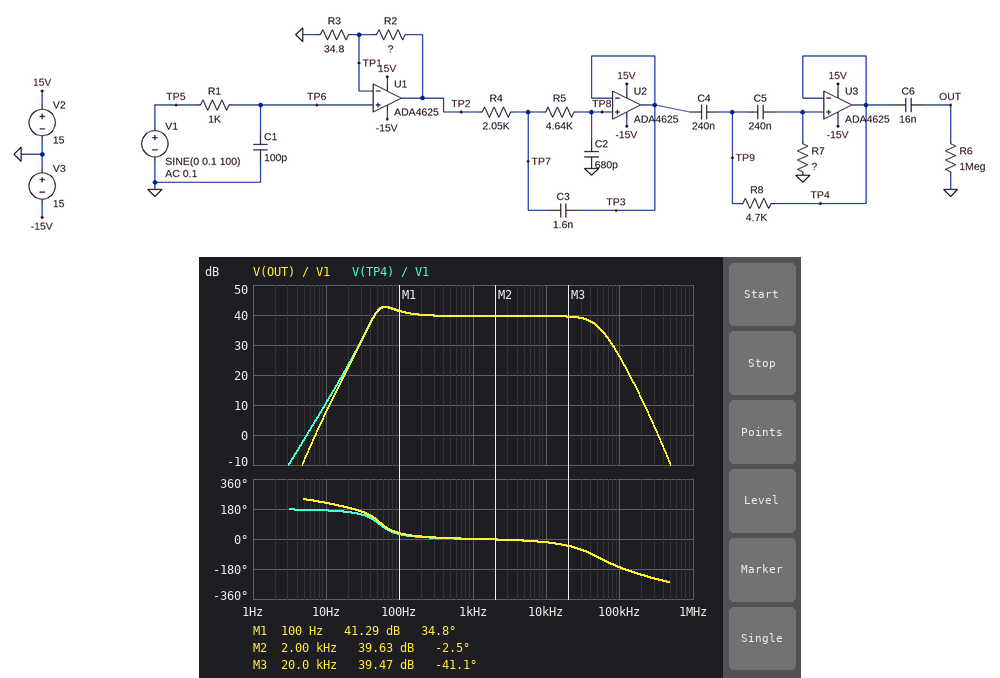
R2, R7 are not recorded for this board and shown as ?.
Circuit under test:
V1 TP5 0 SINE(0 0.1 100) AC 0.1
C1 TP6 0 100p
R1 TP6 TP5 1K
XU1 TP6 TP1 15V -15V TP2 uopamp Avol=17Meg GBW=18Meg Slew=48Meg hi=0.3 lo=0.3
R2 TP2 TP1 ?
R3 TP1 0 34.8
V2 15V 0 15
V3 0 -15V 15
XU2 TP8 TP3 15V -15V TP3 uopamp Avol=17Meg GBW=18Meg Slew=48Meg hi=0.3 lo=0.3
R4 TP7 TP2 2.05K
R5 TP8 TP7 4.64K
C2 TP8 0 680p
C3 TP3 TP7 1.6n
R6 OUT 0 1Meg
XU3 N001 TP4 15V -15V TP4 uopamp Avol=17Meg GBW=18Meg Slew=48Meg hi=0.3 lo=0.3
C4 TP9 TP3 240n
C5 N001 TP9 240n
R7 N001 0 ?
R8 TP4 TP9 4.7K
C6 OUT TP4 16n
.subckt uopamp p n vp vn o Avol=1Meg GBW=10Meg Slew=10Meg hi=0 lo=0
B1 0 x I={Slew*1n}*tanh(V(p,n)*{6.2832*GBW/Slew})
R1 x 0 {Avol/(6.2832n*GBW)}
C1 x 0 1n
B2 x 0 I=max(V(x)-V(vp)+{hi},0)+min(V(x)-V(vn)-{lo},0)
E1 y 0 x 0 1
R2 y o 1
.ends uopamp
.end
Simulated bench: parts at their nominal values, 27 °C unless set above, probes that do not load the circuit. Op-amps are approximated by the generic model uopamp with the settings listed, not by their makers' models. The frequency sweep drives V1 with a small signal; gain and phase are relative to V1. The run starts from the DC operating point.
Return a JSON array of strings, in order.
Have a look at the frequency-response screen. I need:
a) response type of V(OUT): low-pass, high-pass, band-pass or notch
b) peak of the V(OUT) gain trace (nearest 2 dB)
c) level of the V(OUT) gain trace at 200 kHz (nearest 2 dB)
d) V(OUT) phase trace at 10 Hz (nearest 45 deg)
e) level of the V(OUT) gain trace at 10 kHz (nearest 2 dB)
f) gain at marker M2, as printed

["band-pass", "42 dB", "12 dB", "225 deg", "40 dB", "39.63 dB"]
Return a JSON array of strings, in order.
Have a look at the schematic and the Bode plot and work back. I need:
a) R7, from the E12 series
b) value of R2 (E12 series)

["33 kΩ", "3.3 kΩ"]
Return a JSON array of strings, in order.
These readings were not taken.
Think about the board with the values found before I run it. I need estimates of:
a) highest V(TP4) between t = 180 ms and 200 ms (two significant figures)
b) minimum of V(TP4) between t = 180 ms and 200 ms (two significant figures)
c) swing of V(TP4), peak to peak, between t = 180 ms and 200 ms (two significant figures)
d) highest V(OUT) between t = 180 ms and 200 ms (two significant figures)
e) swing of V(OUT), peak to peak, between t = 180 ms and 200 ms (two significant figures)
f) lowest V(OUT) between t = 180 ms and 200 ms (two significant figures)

["12 V", "-12 V", "23 V", "12 V", "23 V", "-12 V"]
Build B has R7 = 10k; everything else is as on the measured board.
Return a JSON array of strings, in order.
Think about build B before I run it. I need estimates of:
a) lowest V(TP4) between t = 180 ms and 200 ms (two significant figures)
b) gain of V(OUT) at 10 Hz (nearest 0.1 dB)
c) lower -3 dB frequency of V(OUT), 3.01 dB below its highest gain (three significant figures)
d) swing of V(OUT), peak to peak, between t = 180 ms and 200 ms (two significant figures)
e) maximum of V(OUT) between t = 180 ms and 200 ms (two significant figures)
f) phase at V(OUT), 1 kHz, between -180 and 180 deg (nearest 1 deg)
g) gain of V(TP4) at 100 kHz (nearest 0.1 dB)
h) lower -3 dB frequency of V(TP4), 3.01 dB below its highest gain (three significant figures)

["-7.2 V", "-2.8 dB", "94.5 Hz", "14 V", "7.2 V", "6 deg", "26.0 dB", "94.0 Hz"]
